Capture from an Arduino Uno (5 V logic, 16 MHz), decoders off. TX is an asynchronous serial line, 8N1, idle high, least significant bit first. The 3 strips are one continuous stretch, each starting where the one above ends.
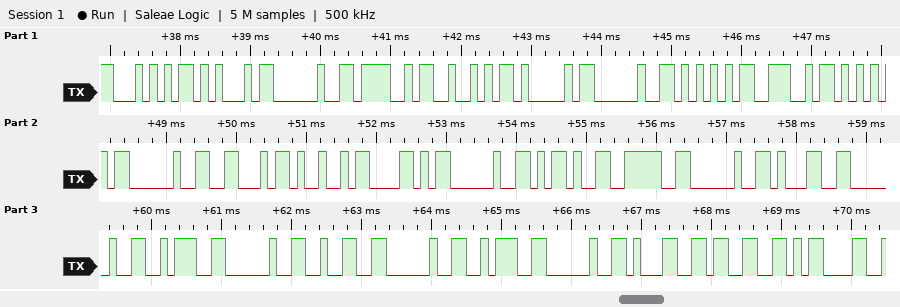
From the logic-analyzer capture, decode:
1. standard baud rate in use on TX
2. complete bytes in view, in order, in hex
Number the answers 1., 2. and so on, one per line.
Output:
1. 9600 baud
2. 54 45 20 4F 52 41 20 55 4E 55 20 46 49 58 20 2D 3E 20 31 20 3A 20 32 20 3A 20 31 33 0D
